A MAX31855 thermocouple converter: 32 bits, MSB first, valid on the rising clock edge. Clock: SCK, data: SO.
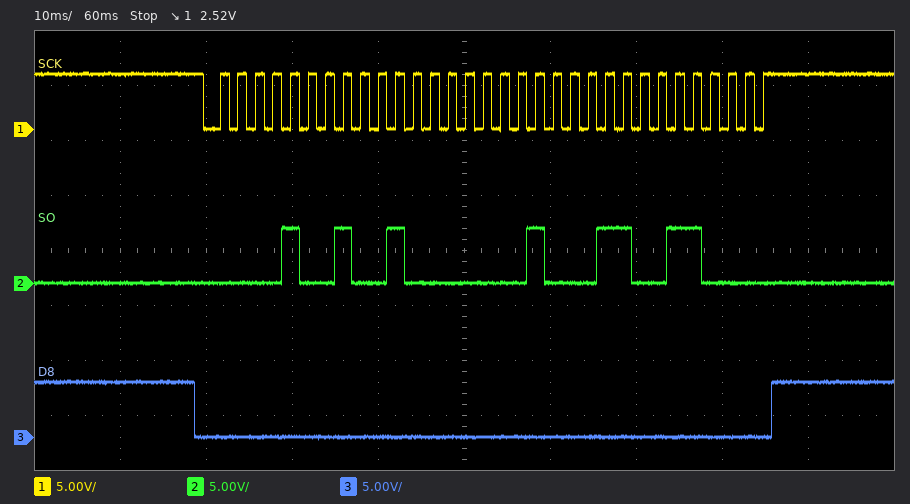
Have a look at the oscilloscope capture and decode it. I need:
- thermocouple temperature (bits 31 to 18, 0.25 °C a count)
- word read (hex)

146.00 °C
0x09202330
